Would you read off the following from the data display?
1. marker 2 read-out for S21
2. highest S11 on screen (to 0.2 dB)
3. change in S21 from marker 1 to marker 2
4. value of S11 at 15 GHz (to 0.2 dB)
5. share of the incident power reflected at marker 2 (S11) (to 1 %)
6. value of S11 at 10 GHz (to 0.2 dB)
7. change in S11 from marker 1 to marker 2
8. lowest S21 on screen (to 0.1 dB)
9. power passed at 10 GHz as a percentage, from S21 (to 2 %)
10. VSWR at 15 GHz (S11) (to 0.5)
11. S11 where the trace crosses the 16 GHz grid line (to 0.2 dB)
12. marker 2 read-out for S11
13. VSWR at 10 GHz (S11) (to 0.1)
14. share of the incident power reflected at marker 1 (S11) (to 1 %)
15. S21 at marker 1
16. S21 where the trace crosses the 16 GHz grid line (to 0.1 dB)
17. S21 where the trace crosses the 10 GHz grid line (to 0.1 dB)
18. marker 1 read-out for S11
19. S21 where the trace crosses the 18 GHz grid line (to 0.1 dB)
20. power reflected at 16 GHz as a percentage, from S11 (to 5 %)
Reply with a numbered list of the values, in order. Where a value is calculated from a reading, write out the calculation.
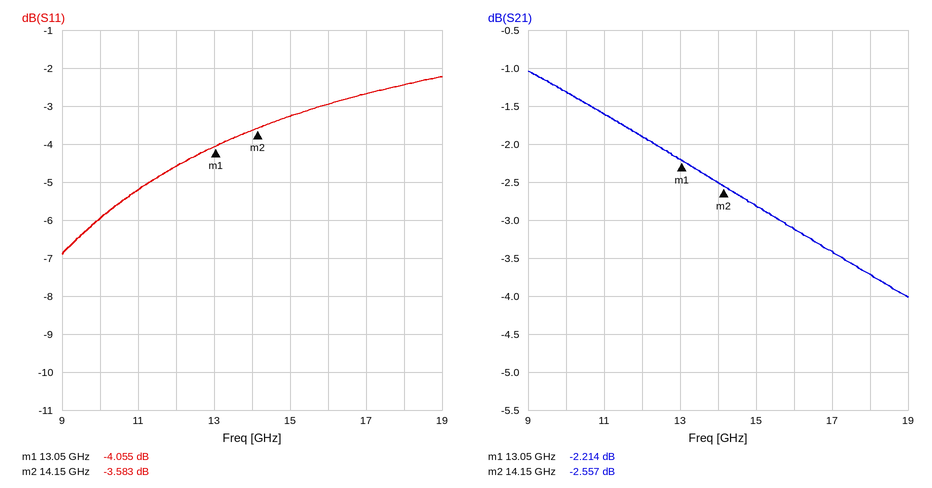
1. -2.557 dB
2. -2.2 dB
3. -2.557 − (-2.214) = -0.343 dB
4. -3.2 dB
5. 10^(-3.583/10) ≈ 44 %
6. -6.0 dB
7. -3.583 − (-4.055) = 0.472 dB
8. -4.0 dB
9. 10^(-1.3/10) ≈ 74 %
10. |Γ| = 10^(-3.2/20) = 0.6918; VSWR = (1 + 0.6918)/(1 − 0.6918) ≈ 5.5
11. -3.0 dB
12. -3.583 dB
13. |Γ| = 10^(-6/20) = 0.5012; VSWR = (1 + 0.5012)/(1 − 0.5012) ≈ 3.0
14. 10^(-4.055/10) ≈ 39 %
15. -2.214 dB
16. -3.1 dB
17. -1.3 dB
18. -4.055 dB
19. -3.7 dB
20. 10^(-3/10) ≈ 50 %
